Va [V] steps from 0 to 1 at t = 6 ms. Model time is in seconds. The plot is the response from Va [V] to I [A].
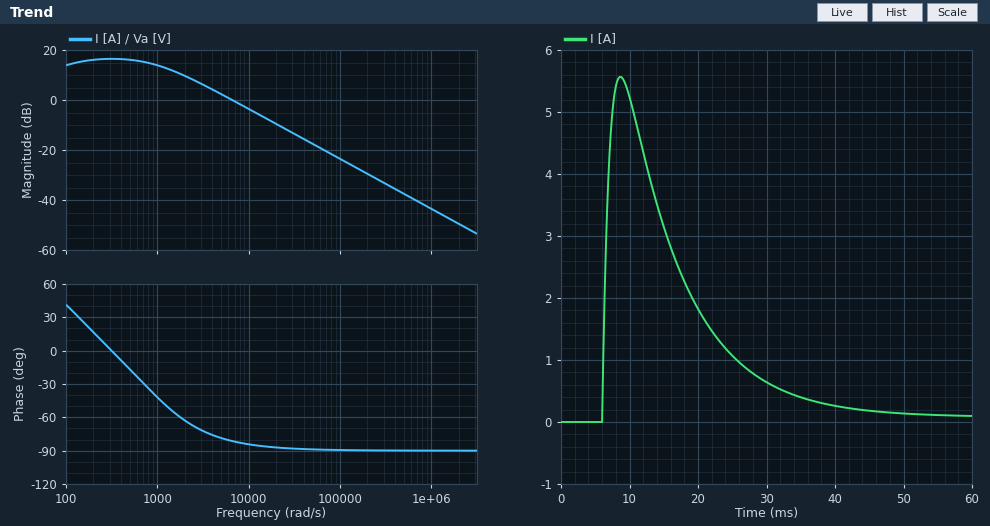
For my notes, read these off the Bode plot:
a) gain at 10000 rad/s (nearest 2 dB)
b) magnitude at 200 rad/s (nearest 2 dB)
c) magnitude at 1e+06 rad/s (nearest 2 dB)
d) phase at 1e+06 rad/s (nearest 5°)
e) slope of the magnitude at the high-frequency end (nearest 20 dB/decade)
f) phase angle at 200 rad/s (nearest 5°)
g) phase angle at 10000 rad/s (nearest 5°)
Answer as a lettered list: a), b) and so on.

a) -4 dB
b) 16 dB
c) -44 dB
d) -90°
e) -20 dB/decade
f) 15°
g) -85°
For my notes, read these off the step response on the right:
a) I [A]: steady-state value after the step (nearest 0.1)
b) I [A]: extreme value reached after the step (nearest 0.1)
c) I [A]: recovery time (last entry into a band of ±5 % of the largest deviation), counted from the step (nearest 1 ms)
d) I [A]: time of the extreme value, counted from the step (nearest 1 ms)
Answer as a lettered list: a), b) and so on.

a) 0.1
b) 5.6
c) 30 ms
d) 3 ms
